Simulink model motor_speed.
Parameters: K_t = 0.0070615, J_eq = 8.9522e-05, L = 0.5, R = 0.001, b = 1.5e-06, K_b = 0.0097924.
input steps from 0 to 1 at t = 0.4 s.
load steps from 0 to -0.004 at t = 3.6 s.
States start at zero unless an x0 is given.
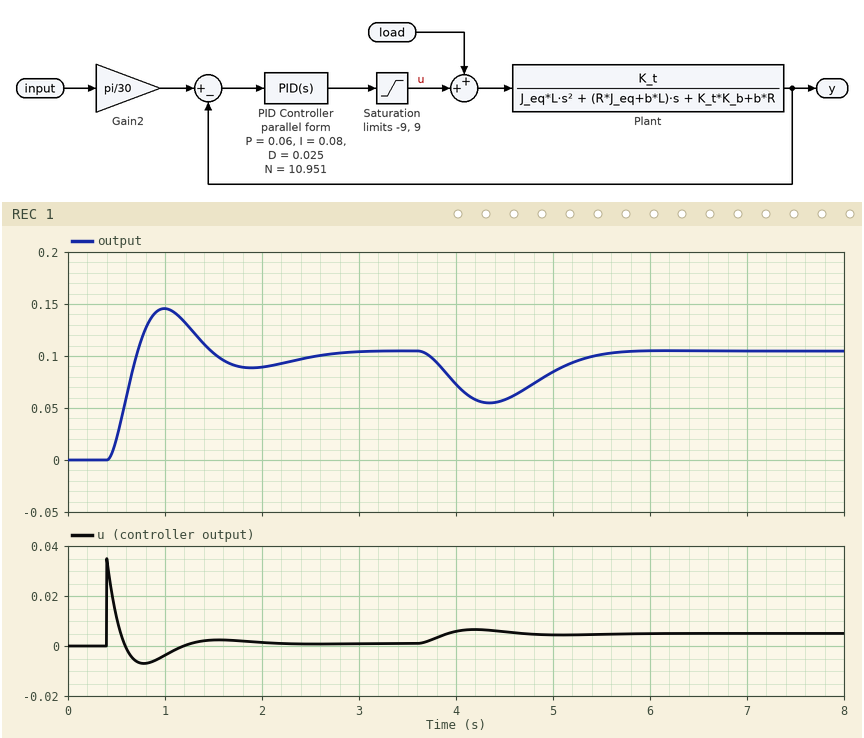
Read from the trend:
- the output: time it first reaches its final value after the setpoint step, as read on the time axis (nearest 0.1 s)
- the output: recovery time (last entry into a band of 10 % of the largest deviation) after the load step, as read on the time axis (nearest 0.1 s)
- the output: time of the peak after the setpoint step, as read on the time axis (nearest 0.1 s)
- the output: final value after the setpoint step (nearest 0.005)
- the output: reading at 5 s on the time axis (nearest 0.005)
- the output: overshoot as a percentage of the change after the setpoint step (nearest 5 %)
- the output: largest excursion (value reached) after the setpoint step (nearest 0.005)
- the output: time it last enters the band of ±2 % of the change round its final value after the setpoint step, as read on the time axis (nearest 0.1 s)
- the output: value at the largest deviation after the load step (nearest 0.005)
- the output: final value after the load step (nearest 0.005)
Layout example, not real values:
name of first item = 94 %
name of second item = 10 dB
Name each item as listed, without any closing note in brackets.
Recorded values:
the output: time it first reaches its final value after the setpoint step, as read on the time axis = 0.7 s
the output: recovery time (last entry into a band of 10 % of the largest deviation) after the load step, as read on the time axis = 5.4 s
the output: time of the peak after the setpoint step, as read on the time axis = 1.0 s
the output: final value after the setpoint step = 0.105
the output: reading at 5 s on the time axis = 0.085
the output: overshoot as a percentage of the change after the setpoint step = 40 %
the output: largest excursion (value reached) after the setpoint step = 0.145
the output: time it last enters the band of ±2 % of the change round its final value after the setpoint step, as read on the time axis = 2.8 s
the output: value at the largest deviation after the load step = 0.055
the output: final value after the load step = 0.105
